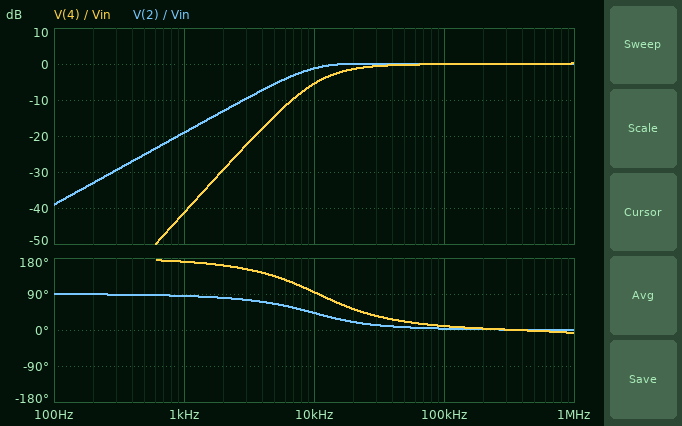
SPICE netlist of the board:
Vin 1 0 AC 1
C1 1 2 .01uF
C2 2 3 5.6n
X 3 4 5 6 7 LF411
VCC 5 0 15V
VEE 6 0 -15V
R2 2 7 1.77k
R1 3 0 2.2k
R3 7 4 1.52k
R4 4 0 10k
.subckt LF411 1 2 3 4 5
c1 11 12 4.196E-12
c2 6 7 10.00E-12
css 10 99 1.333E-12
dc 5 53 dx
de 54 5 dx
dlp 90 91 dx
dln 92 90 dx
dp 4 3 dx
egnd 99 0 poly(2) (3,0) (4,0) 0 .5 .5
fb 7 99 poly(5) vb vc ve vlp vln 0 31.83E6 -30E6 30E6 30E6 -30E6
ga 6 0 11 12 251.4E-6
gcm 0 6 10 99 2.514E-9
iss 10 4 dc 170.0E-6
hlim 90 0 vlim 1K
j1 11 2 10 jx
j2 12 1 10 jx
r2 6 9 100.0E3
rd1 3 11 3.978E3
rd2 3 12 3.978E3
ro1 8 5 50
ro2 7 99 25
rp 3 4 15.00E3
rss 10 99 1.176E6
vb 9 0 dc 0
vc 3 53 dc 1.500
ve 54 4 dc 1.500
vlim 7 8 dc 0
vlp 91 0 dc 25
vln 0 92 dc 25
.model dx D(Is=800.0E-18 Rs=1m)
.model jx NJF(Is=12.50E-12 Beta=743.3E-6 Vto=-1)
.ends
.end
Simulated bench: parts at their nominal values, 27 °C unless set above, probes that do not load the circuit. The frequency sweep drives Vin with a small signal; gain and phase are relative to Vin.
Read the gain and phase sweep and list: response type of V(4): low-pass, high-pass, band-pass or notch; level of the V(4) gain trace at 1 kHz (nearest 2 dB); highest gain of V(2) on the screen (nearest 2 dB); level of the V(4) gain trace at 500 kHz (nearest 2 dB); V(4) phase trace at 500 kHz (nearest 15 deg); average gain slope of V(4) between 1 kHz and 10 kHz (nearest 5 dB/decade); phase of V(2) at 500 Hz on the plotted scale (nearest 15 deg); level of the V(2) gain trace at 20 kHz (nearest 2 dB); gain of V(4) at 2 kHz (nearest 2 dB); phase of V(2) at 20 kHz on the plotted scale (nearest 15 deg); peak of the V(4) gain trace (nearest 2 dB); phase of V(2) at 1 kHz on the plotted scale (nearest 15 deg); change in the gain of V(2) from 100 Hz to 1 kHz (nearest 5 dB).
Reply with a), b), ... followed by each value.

a) high-pass
b) -42 dB
c) 0 dB
d) 0 dB
e) 0 deg
f) 35 dB/decade
g) 90 deg
h) 0 dB
i) -30 dB
j) 15 deg
k) 0 dB
l) 90 deg
m) 20 dB
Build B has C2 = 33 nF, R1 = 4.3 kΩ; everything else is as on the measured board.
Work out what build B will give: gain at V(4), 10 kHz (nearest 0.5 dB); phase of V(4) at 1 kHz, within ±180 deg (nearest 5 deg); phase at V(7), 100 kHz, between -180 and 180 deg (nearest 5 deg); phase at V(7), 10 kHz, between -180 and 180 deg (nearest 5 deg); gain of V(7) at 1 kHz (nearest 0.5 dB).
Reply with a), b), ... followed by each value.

a) 0.5 dB
b) 160 deg
c) 0 deg
d) 20 deg
e) -18.5 dB
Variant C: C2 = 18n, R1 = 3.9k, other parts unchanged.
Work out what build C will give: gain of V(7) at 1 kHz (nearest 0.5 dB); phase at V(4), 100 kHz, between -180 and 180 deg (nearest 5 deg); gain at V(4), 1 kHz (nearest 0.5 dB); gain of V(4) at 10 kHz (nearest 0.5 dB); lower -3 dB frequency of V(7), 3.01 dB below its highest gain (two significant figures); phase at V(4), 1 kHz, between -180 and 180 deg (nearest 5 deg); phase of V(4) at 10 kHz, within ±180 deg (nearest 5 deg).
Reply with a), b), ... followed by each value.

a) -25.0 dB
b) 0 deg
c) -26.0 dB
d) 0.5 dB
e) 4.5 kHz
f) 165 deg
g) 30 deg
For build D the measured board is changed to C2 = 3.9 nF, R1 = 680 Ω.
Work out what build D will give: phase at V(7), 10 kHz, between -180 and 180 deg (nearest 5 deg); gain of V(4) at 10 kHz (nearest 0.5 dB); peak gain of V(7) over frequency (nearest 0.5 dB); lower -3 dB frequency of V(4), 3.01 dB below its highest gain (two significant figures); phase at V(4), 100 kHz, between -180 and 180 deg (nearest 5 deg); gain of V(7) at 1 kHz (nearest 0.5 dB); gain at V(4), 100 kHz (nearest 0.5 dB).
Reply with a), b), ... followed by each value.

a) 120 deg
b) -19.5 dB
c) 3.5 dB
d) 170 kHz
e) 40 deg
f) -53.5 dB
g) -2.0 dB
